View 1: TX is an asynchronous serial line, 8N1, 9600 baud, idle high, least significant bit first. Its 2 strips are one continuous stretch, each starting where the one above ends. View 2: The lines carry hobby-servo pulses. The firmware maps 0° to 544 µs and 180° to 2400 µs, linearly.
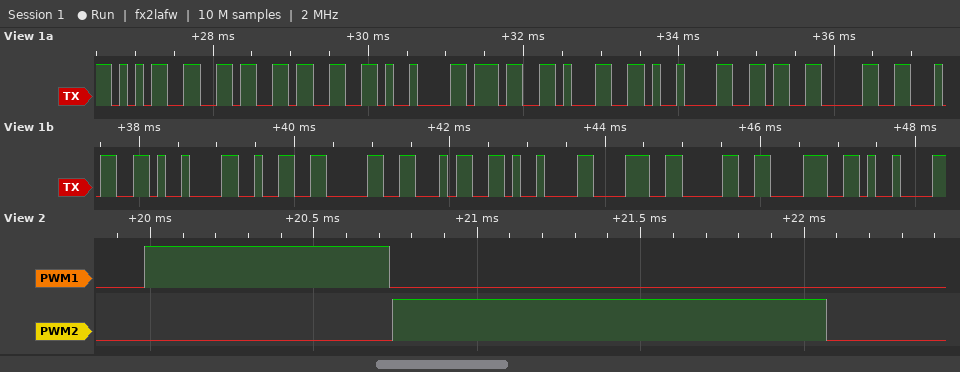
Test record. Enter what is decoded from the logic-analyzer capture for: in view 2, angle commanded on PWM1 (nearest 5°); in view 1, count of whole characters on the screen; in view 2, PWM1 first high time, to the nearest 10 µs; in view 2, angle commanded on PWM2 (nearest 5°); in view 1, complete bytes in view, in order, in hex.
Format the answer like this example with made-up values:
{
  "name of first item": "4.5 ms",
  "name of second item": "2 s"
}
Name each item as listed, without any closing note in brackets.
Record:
{
  "in view 2, angle commanded on PWM1": "20°",
  "in view 1, count of whole characters on the screen": "19",
  "in view 2, PWM1 first high time, to the nearest 10 µs": "750 µs",
  "in view 2, angle commanded on PWM2": "75°",
  "in view 1, complete bytes in view, in order, in hex": "35 36 33 09 37 31 09 36 30 34 09 32 30 34 09 38 30 38 09"
}
